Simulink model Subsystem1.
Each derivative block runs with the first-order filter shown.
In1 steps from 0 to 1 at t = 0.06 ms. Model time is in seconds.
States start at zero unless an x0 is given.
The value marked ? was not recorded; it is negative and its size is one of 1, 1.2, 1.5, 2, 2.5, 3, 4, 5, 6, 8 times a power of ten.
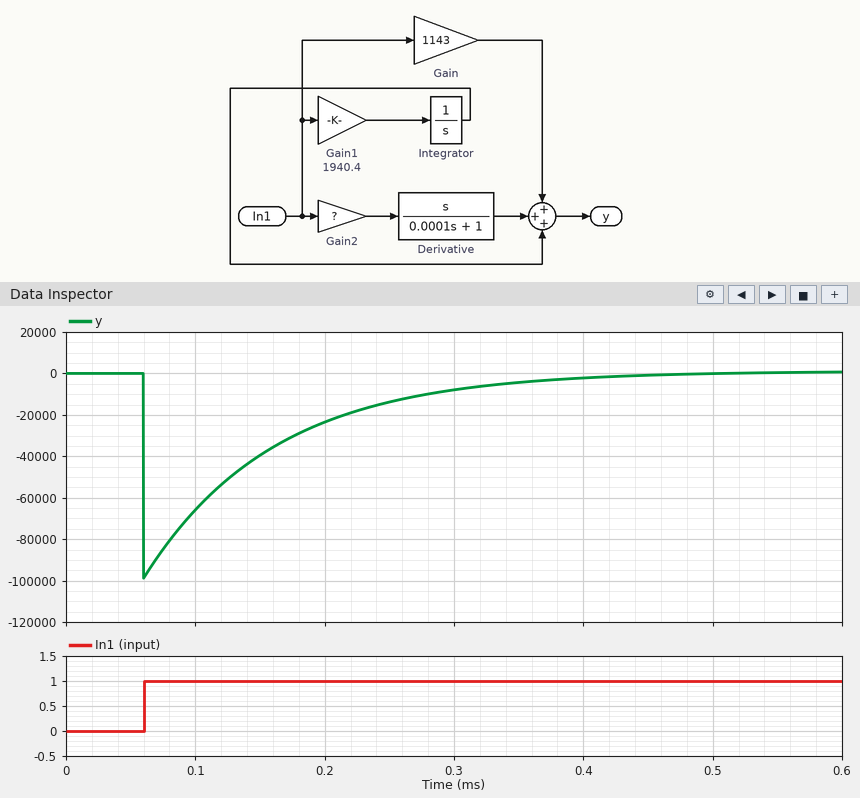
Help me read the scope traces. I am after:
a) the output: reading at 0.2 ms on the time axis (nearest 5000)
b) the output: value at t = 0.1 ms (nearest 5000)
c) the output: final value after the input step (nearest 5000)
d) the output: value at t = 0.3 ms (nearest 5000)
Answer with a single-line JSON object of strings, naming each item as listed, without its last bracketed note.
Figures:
{"the output: reading at 0.2 ms on the time axis": "-25000", "the output: value at t = 0.1 ms": "-65000", "the output: final value after the input step": "0", "the output: value at t = 0.3 ms": "-10000"}
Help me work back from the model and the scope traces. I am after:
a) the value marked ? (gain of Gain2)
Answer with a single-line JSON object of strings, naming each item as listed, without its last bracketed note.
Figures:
{"the value marked ?": "-10"}
